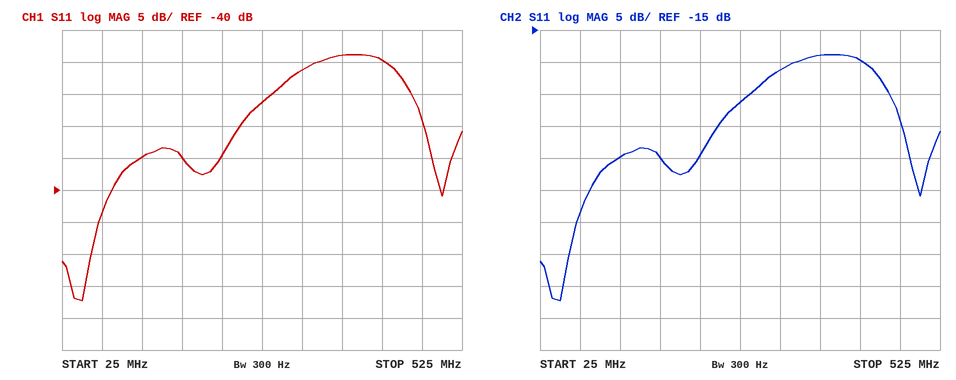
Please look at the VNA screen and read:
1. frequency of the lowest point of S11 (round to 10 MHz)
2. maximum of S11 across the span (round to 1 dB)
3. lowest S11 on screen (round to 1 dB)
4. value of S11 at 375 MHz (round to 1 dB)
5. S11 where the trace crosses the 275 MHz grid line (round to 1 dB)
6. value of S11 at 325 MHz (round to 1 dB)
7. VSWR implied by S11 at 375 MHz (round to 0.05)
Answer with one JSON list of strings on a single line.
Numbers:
["50 MHz", "-19 dB", "-57 dB", "-19 dB", "-26 dB", "-21 dB", "1.25"]
